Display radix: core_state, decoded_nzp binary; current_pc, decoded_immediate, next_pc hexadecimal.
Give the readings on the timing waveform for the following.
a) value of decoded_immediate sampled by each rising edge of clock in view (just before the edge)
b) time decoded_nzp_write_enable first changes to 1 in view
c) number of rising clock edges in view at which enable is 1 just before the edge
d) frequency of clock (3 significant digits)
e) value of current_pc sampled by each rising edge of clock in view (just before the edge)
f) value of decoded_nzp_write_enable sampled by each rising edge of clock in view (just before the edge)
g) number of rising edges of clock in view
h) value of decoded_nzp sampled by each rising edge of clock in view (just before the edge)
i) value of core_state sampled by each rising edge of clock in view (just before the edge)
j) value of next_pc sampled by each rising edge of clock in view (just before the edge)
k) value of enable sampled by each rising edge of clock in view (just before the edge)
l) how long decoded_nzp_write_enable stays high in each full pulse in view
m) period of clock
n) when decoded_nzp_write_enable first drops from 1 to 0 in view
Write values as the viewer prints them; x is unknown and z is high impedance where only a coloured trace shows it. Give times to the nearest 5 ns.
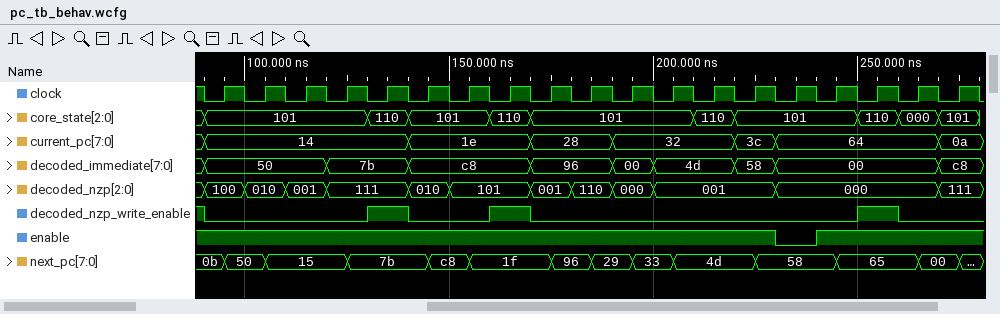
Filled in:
50, 50, 50, 7b, 7b, c8, c8, c8, 96, 96, 00, 4d, 4d, 58, 00, 00, 00, 00, c8
130 ns
18
100 MHz
14, 14, 14, 14, 14, 1e, 1e, 1e, 28, 28, 32, 32, 32, 3c, 64, 64, 64, 64, 0a
0 0 0 0 1 0 0 1 0 0 0 0 0 0 0 0 1 0 0
19
100, 010, 001, 111, 111, 010, 101, 101, 001, 110, 000, 001, 001, 001, 000, 000, 000, 000, 111
101, 101, 101, 101, 110, 101, 101, 110, 101, 101, 101, 101, 110, 101, 101, 101, 110, 000, 101
0b, 50, 15, 15, 7b, 7b, c8, 1f, 1f, 96, 29, 33, 4d, 4d, 58, 58, 65, 65, 00
1 1 1 1 1 1 1 1 1 1 1 1 1 1 0 1 1 1 1
10 ns, 10 ns, 10 ns
10 ns
90 ns
